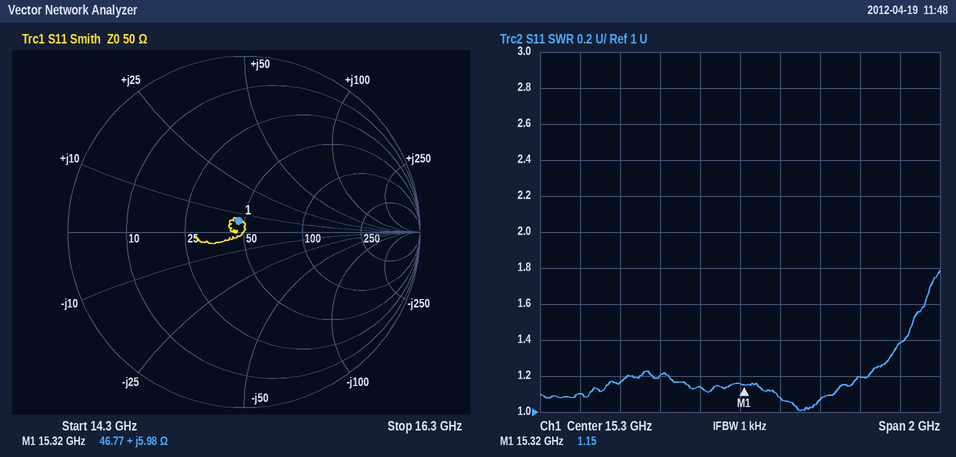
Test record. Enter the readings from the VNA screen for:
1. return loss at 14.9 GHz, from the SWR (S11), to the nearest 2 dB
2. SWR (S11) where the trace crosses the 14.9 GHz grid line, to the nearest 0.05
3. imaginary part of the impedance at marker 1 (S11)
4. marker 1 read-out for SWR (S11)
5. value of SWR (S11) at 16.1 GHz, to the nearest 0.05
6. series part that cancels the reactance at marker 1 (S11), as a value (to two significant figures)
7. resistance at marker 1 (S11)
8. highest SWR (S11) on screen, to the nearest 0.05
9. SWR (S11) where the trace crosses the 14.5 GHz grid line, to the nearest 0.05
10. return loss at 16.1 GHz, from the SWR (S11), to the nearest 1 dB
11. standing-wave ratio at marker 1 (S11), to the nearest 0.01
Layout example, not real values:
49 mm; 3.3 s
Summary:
20 dB; 1.20; +5.98 Ω; 1.15; 1.40; 1.7 pF; 46.77 Ω; 1.80; 1.10; 16 dB; 1.15
